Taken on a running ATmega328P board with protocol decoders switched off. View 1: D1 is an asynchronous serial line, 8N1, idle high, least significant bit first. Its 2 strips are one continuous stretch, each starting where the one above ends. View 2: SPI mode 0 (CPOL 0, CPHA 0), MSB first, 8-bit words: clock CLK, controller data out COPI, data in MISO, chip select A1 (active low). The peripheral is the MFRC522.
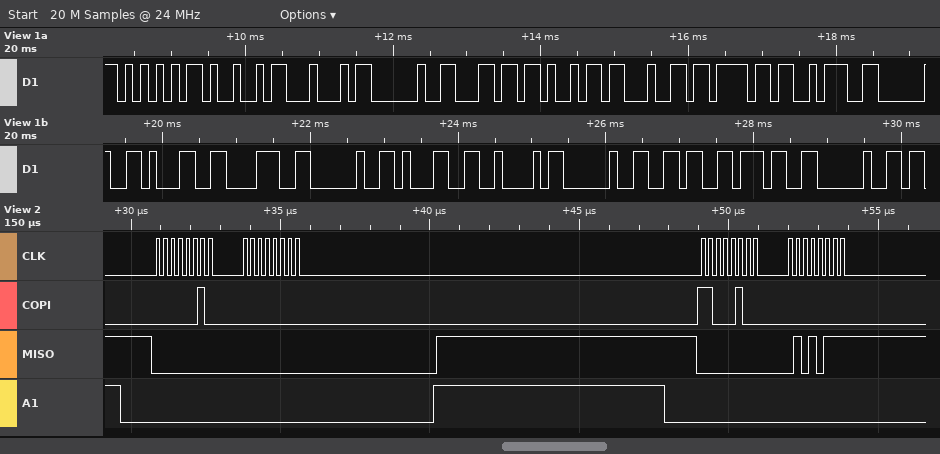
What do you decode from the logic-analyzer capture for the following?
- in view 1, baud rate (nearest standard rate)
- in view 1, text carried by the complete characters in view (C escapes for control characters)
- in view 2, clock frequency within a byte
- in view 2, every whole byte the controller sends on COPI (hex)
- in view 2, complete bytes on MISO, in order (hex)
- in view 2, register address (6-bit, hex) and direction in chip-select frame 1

9600 baud
"UID lido: 18 1B 67 "
4 MHz
02 00 C4 00
00 00 00 57
0x01 write
